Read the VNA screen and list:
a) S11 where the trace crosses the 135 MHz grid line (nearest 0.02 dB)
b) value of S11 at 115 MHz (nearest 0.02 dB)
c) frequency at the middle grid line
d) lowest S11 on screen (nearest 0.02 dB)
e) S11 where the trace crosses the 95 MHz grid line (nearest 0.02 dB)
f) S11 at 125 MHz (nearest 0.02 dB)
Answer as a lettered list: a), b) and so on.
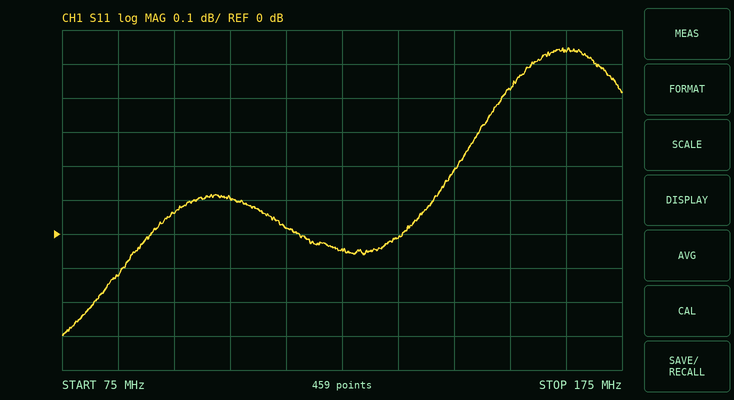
a) -0.02 dB
b) 0.02 dB
c) 125 MHz
d) -0.30 dB
e) 0.06 dB
f) -0.04 dB
